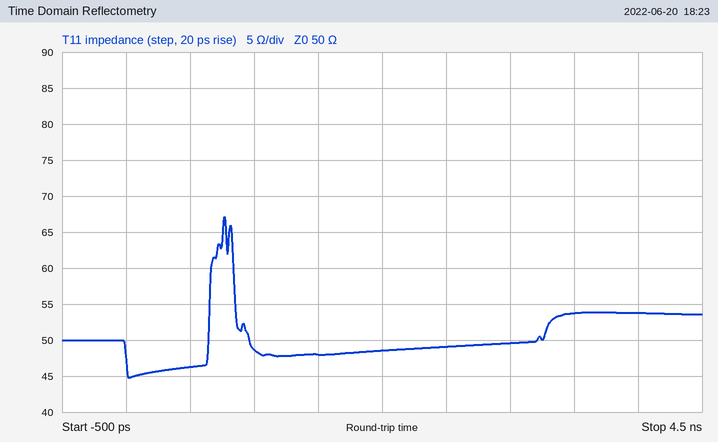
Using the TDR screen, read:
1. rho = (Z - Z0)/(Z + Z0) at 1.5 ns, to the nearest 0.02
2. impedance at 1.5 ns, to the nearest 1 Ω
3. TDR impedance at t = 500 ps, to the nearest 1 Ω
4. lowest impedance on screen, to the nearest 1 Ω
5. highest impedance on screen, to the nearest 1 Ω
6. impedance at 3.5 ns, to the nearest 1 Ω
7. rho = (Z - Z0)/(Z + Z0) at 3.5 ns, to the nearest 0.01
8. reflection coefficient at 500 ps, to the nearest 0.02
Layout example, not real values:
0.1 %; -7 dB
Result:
-0.02; 48 Ω; 46 Ω; 45 Ω; 67 Ω; 54 Ω; +0.04; -0.04
